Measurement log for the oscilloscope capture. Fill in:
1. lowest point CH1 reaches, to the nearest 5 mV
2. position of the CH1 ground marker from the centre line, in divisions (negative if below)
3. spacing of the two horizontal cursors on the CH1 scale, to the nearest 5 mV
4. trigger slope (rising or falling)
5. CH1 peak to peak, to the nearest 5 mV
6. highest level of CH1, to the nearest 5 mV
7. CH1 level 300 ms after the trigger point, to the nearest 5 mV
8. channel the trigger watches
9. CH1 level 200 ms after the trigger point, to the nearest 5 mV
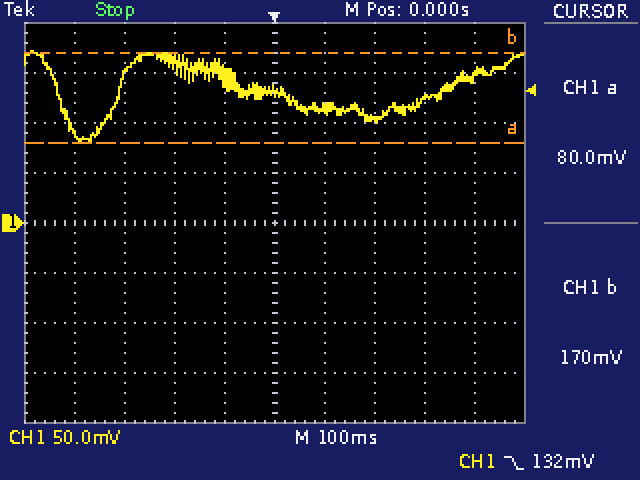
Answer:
80 mV
0.0 div
90 mV
falling
90 mV
170 mV
125 mV
CH1
105 mV
